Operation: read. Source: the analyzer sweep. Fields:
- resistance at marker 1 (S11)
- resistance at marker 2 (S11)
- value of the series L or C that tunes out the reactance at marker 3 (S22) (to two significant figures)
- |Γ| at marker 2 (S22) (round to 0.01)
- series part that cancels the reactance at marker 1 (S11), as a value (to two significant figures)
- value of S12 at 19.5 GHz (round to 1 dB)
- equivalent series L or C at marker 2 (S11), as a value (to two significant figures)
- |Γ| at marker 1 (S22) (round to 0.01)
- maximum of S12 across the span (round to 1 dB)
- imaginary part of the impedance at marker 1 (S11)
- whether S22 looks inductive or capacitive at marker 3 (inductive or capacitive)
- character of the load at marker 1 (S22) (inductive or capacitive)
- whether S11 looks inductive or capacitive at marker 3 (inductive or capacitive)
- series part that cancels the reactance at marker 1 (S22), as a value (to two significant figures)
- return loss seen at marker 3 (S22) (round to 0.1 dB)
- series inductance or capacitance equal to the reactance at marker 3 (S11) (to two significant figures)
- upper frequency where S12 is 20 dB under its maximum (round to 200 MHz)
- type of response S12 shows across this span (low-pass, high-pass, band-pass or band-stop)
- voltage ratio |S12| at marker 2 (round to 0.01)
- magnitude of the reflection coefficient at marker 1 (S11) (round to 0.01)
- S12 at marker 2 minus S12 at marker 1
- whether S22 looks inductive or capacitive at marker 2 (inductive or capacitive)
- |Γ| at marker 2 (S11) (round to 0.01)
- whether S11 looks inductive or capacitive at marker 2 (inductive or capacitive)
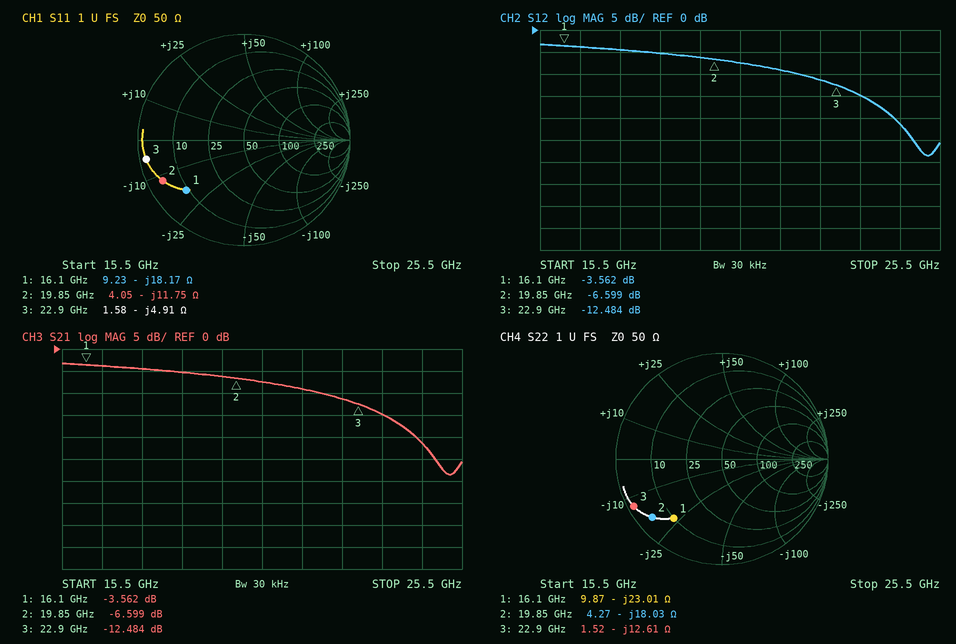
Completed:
9.23 Ω
4.05 Ω
88 pH
0.86
180 pH
-6 dB
680 fF
0.72
-3 dB
-18.17 Ω
capacitive
capacitive
capacitive
230 pH
0.5 dB
1.4 pF
24.6 GHz
low-pass
0.47
0.72
-3.037 dB
capacitive
0.86
capacitive
